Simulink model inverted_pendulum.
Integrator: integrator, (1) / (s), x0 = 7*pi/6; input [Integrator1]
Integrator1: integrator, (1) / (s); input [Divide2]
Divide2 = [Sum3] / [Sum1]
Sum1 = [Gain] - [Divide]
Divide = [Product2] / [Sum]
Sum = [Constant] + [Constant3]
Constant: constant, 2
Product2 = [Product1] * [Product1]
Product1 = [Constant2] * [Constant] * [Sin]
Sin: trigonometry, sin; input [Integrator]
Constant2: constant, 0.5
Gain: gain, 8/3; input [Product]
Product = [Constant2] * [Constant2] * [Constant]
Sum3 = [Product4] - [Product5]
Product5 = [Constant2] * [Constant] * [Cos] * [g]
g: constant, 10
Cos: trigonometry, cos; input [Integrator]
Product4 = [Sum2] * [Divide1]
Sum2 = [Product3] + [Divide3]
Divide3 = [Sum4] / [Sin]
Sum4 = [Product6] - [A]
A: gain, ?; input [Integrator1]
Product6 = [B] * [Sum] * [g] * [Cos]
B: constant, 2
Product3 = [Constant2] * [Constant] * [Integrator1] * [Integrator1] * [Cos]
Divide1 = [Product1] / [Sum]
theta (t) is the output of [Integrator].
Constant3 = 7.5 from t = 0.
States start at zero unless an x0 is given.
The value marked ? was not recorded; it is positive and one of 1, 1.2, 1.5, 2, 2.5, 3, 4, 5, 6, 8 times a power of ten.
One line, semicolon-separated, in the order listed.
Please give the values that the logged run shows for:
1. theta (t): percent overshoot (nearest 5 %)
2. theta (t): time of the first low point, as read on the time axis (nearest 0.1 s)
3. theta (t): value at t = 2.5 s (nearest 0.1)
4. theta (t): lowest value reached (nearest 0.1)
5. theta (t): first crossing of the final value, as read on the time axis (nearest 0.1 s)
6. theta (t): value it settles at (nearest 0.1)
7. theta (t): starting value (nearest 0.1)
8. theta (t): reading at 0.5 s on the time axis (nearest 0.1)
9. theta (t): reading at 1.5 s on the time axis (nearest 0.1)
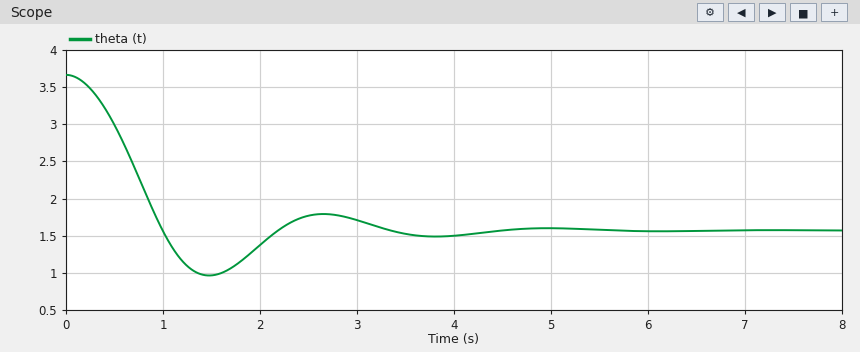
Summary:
30 %; 1.5 s; 1.8; 1.0; 1.0 s; 1.6; 3.7; 3.0; 1.0
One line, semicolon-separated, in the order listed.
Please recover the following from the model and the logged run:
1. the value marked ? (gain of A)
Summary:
20
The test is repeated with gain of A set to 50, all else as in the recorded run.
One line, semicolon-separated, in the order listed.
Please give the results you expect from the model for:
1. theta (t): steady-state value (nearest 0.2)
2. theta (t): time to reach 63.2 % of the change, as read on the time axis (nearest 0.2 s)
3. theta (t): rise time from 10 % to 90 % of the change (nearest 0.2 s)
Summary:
1.6; 1.0 s; 1.2 s
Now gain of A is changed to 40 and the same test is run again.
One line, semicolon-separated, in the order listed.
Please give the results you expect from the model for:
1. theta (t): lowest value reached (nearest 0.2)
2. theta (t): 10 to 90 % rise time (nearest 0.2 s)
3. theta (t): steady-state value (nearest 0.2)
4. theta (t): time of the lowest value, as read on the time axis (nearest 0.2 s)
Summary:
1.4; 1.0 s; 1.6; 1.8 s
